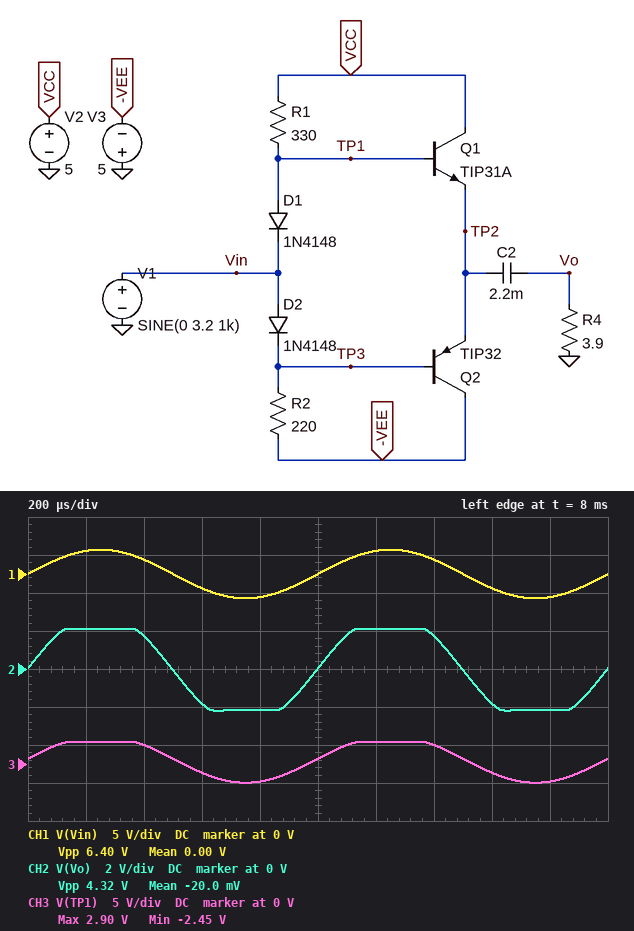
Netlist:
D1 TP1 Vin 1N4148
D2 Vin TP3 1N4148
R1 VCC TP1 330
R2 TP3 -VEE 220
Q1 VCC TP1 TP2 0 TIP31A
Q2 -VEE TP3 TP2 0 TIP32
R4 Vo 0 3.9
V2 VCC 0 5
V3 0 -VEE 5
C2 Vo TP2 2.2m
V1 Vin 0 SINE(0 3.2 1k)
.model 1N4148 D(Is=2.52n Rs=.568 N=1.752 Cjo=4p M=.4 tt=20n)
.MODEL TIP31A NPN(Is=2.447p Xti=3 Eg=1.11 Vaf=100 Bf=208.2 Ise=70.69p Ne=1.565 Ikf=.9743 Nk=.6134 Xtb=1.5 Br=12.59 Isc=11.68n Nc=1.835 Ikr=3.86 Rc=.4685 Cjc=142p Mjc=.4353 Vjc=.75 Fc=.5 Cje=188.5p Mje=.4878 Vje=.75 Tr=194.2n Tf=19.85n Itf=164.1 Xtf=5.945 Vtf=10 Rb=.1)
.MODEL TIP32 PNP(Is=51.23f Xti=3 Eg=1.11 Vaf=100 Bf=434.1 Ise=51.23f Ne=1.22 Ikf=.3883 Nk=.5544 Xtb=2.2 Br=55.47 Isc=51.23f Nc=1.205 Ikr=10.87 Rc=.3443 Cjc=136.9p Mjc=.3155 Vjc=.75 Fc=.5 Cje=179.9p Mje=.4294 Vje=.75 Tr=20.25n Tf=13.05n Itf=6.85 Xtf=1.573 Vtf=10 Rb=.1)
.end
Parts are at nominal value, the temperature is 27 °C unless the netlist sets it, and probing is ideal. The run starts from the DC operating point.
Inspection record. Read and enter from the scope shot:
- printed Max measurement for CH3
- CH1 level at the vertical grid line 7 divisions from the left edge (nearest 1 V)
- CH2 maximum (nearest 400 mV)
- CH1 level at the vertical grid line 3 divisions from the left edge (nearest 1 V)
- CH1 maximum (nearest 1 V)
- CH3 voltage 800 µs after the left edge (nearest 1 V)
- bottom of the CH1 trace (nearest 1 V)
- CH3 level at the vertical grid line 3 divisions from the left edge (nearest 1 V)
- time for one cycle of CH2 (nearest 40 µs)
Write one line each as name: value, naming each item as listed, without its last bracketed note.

printed Max measurement for CH3: 2.90 V
CH1 level at the vertical grid line 7 divisions from the left edge: 2 V
CH2 maximum: 2.0 V
CH1 level at the vertical grid line 3 divisions from the left edge: -2 V
CH1 maximum: 3 V
CH3 voltage 800 µs after the left edge: -2 V
bottom of the CH1 trace: -3 V
CH3 level at the vertical grid line 3 divisions from the left edge: -1 V
time for one cycle of CH2: 1.00 ms
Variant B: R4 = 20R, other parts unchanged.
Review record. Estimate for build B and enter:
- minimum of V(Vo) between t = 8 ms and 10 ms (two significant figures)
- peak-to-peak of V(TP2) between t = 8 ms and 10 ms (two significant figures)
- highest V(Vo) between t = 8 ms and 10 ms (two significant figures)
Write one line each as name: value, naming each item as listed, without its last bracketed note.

minimum of V(Vo) between t = 8 ms and 10 ms: -3.1 V
peak-to-peak of V(TP2) between t = 8 ms and 10 ms: 6.2 V
highest V(Vo) between t = 8 ms and 10 ms: 3.1 V
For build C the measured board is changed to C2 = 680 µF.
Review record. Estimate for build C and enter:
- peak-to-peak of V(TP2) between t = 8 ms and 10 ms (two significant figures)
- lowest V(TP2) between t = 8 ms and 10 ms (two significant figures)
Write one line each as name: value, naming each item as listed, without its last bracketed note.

peak-to-peak of V(TP2) between t = 8 ms and 10 ms: 4.4 V
lowest V(TP2) between t = 8 ms and 10 ms: -2.2 V
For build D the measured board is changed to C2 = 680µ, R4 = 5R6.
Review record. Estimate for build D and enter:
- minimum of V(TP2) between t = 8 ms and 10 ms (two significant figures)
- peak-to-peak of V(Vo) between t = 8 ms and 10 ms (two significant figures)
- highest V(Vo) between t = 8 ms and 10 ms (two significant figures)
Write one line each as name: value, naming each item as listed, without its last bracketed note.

minimum of V(TP2) between t = 8 ms and 10 ms: -2.6 V
peak-to-peak of V(Vo) between t = 8 ms and 10 ms: 5.2 V
highest V(Vo) between t = 8 ms and 10 ms: 2.6 V
